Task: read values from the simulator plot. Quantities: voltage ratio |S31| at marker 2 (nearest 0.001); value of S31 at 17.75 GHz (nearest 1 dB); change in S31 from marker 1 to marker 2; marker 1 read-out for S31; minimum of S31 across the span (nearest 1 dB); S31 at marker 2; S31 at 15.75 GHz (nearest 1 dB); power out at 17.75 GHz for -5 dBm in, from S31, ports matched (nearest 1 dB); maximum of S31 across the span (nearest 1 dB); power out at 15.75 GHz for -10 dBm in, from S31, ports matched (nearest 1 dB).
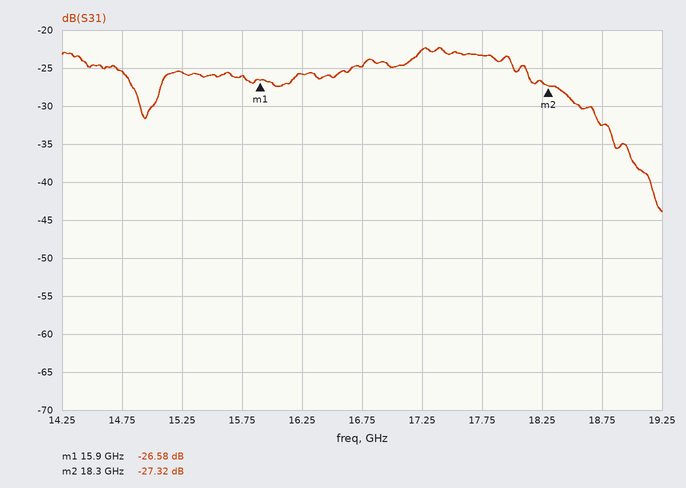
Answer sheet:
0.043
-23 dB
-0.74 dB
-26.58 dB
-44 dB
-27.32 dB
-26 dB
-28 dBm
-22 dB
-36 dBm
